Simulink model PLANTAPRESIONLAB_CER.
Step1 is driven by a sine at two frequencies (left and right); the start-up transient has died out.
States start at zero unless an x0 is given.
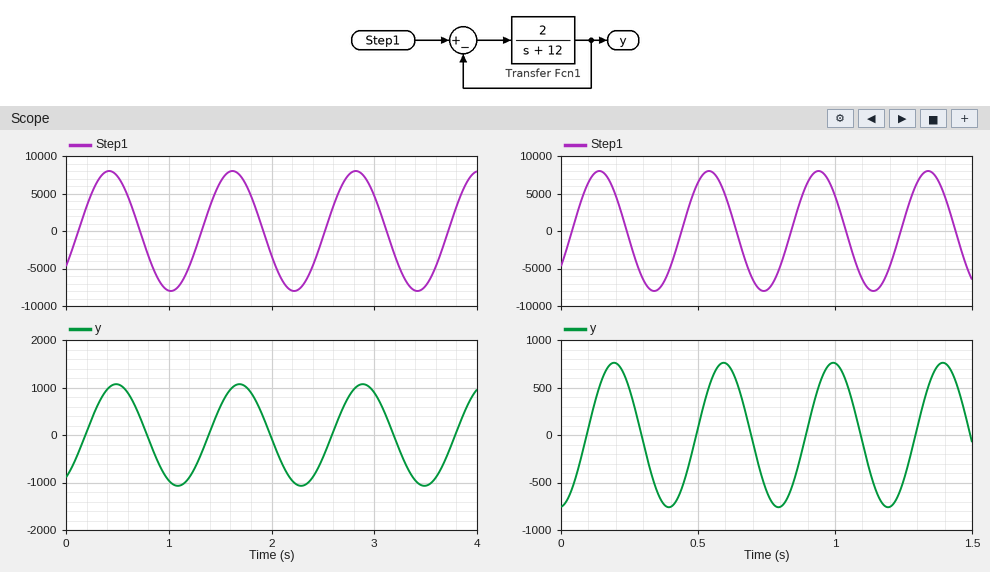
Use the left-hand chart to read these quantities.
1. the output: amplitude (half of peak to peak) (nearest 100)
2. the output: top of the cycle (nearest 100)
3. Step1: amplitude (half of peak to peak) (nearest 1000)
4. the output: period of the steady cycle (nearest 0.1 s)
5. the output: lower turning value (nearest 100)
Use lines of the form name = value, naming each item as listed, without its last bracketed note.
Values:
the output: amplitude (half of peak to peak) = 1100
the output: top of the cycle = 1100
Step1: amplitude (half of peak to peak) = 8000
the output: period of the steady cycle = 1.2 s
the output: lower turning value = -1100
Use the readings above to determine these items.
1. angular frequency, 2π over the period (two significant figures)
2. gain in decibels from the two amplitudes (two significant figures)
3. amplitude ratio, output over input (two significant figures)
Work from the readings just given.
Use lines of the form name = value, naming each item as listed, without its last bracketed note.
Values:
angular frequency, 2π over the period = 5.2 rad/s
gain in decibels from the two amplitudes = -17 dB
amplitude ratio, output over input = 0.14
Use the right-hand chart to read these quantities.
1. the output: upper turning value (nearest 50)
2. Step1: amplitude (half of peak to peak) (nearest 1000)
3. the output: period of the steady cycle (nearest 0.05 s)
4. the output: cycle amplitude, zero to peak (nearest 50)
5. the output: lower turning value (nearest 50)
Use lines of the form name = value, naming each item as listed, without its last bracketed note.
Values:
the output: upper turning value = 750
Step1: amplitude (half of peak to peak) = 8000
the output: period of the steady cycle = 0.40 s
the output: cycle amplitude, zero to peak = 750
the output: lower turning value = -750
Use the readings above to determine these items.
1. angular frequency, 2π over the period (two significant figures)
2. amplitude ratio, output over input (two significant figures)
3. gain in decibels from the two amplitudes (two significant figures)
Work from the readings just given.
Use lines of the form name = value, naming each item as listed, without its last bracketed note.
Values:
angular frequency, 2π over the period = 16 rad/s
amplitude ratio, output over input = 0.094
gain in decibels from the two amplitudes = -21 dB
